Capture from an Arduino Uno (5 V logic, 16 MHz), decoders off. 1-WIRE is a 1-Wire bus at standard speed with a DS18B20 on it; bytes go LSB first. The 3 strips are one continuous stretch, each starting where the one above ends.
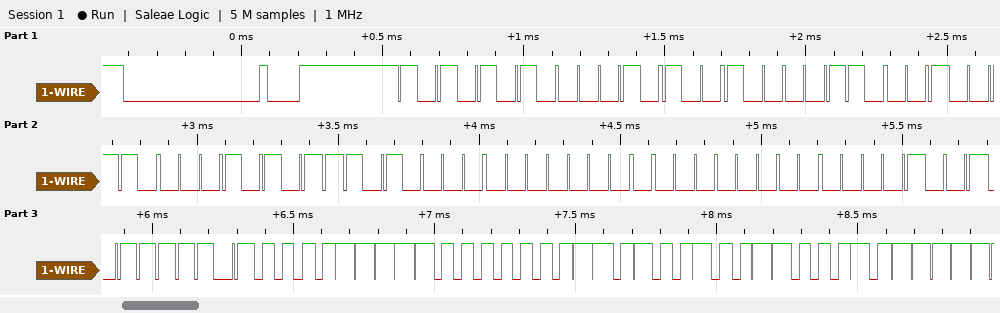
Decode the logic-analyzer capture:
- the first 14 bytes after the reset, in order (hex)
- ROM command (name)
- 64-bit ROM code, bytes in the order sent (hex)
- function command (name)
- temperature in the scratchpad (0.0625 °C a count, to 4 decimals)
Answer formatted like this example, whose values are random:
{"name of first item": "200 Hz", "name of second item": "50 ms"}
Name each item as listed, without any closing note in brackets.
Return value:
{"the first 14 bytes after the reset, in order": "55 28 61 64 A8 0B 00 00 90 BE F0 01 4B 46", "ROM command": "Match ROM", "64-bit ROM code, bytes in the order sent": "28 61 64 A8 0B 00 00 90", "function command": "Read Scratchpad", "temperature in the scratchpad": "31.0000 °C"}
